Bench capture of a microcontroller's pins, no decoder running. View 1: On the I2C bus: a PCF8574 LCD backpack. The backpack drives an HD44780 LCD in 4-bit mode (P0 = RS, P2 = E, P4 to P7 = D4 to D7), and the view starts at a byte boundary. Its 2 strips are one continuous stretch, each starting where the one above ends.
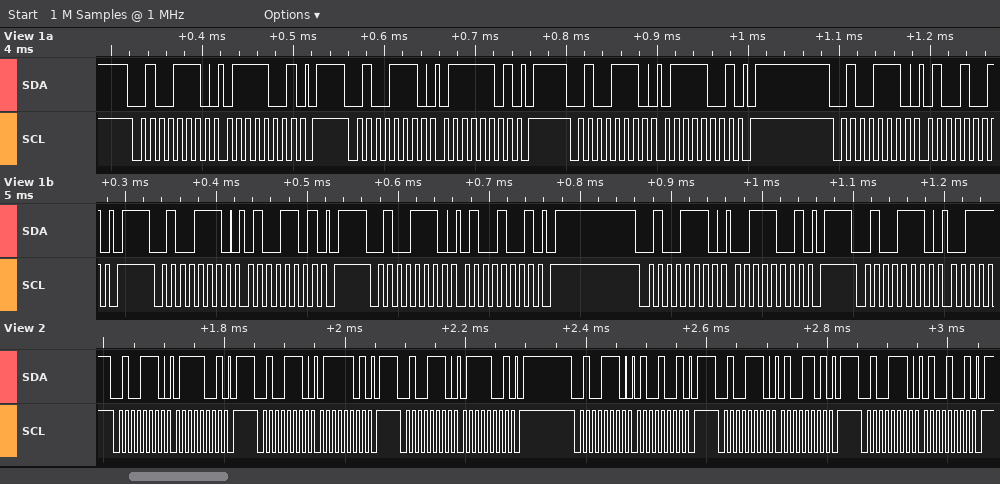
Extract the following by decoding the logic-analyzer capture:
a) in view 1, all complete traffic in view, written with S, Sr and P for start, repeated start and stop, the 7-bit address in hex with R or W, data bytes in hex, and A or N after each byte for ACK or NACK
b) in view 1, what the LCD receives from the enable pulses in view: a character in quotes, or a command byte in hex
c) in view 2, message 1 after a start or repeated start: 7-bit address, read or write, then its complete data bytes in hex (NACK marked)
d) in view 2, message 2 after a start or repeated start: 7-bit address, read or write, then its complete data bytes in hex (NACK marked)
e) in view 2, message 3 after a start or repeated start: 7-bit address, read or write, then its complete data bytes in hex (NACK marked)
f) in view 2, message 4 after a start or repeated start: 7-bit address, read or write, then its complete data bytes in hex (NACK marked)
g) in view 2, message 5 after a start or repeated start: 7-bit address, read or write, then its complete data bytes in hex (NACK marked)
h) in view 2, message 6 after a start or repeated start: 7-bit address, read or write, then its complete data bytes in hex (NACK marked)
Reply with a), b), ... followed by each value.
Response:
a) S 27W A 79 A P S 27W A 7D A P S 27W A 79 A P S 27W A 49 A P S 27W A 4D A P S 27W A 49 A P S 27W A 39 A P S 27W A
b) 't'
c) 0x27 write: 79
d) 0x27 write: 7D
e) 0x27 write: 79
f) 0x27 write: 49
g) 0x27 write: 4D
h) 0x27 write: 49
